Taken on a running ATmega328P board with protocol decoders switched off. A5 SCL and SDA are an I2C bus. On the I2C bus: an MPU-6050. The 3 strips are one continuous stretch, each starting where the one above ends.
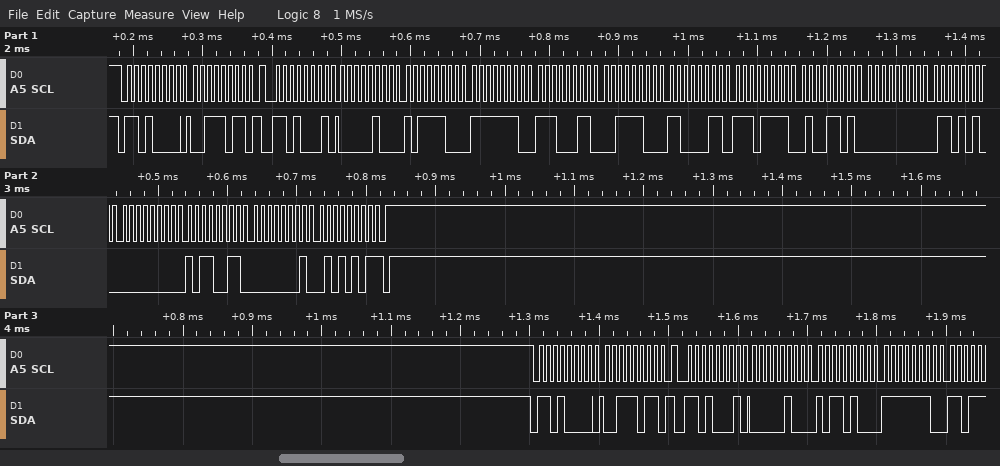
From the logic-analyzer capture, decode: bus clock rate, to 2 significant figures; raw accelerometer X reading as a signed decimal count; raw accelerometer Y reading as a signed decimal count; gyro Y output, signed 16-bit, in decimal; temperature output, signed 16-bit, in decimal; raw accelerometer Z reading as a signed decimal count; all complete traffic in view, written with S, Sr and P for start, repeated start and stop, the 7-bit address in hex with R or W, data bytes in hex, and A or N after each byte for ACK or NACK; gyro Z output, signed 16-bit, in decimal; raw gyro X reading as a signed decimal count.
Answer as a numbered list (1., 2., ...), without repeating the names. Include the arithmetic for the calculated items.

1. 100 kHz
2. 0x04BC = 1212
3. 0xFEE3 = -285
4. 0x00B3 = 179
5. 0xEF4D = -4275
6. 0x3CC3 = 15555
7. S 68W A 3B A Sr 68R A 04 A BC A FE A E3 A 3C A C3 A EF A 4D A 00 A 6A A 00 A B3 A 01 A 55 N P S 68W A 3B A Sr 68R A 04 A B4 A FE A
8. 0x0155 = 341
9. 0x006A = 106
